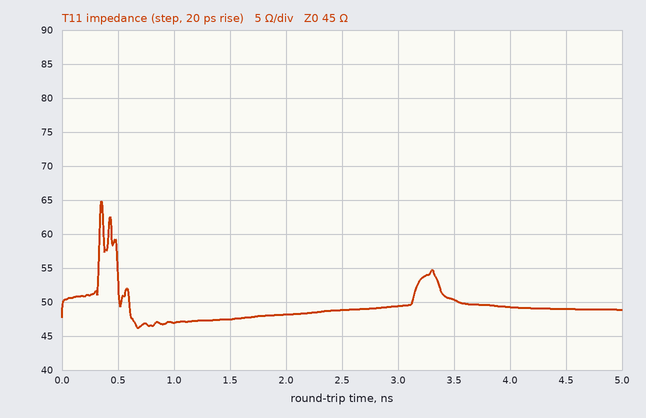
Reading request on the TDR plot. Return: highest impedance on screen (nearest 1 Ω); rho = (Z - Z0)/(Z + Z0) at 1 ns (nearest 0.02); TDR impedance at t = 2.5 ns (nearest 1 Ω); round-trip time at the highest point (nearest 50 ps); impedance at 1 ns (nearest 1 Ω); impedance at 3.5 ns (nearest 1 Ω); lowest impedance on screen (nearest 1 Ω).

65 Ω
+0.02
49 Ω
350 ps
47 Ω
50 Ω
46 Ω
